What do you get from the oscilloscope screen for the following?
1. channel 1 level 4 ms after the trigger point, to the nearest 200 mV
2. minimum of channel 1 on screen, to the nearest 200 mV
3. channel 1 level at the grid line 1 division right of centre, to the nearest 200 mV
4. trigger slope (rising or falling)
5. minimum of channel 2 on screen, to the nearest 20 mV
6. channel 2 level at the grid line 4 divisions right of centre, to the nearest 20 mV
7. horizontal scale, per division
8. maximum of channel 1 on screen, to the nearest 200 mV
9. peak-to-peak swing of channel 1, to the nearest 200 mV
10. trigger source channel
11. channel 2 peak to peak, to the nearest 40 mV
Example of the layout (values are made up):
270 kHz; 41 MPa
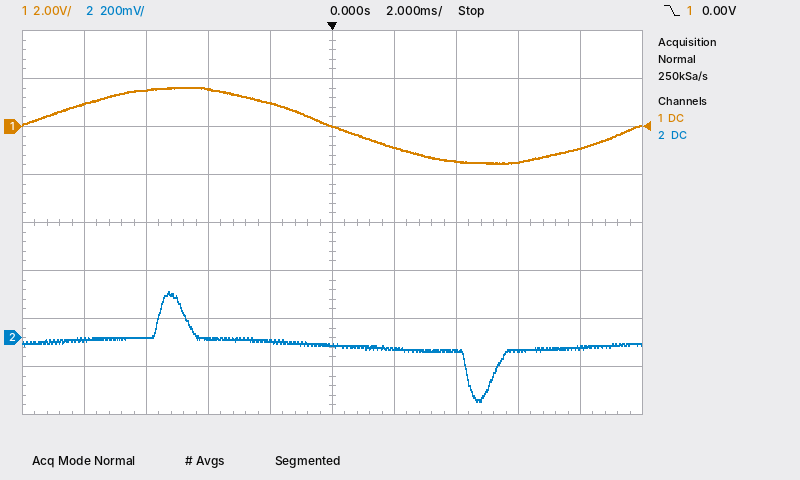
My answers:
-1.4 V; -1.6 V; -800 mV; falling; -260 mV; -40 mV; 2 ms; 1.6 V; 3.2 V; channel 1; 440 mV
